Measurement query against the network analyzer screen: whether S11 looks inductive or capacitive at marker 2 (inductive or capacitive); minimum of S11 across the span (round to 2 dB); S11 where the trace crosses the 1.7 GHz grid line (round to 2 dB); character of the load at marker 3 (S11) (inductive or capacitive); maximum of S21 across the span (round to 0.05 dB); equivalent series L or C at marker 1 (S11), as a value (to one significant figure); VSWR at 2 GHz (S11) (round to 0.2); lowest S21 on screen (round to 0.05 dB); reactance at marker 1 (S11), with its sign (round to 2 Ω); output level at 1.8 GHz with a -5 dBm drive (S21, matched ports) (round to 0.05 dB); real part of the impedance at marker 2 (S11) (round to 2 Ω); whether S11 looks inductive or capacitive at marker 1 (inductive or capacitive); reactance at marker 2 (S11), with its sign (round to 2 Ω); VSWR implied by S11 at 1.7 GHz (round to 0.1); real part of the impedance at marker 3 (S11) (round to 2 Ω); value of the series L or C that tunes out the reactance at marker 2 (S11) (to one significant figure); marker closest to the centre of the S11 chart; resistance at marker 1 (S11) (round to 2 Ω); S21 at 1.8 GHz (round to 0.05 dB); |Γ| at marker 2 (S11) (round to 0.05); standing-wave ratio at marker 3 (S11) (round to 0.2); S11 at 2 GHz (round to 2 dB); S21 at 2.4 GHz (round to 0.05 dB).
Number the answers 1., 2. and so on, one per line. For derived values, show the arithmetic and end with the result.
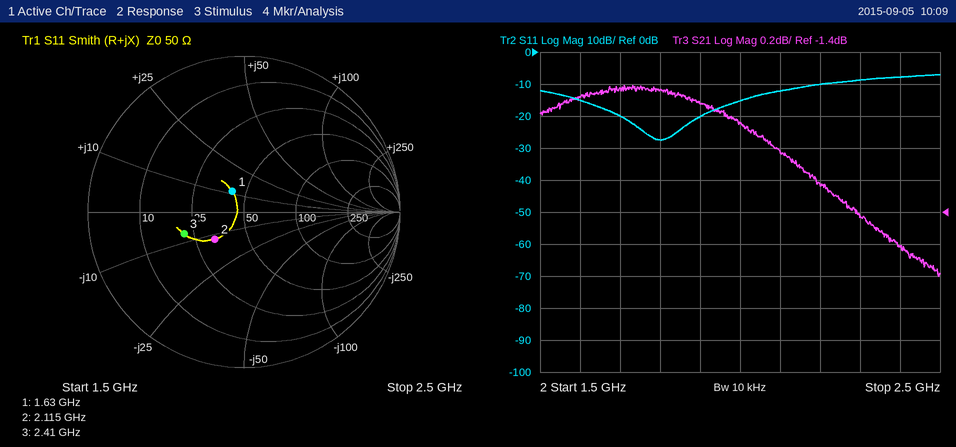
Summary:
1. capacitive
2. -28 dB
3. -20 dB
4. capacitive
5. -0.60 dB
6. L = 12 Ω/(2π × 1.63 GHz) ≈ 1 nH
7. |Γ| = 10^(-16/20) = 0.1585; VSWR = (1 + 0.1585)/(1 − 0.1585) ≈ 1.4
8. -1.80 dB
9. +12 Ω
10. -5 dBm + (-0.65 dB) = -5.65 dBm
11. 32 Ω
12. inductive
13. -12 Ω
14. |Γ| = 10^(-20/20) = 0.1000; VSWR = (1 + 0.1000)/(1 − 0.1000) ≈ 1.2
15. 22 Ω
16. L = 12 Ω/(2π × 2.115 GHz) ≈ 903 pH, so 900 pH to one significant figure
17. marker 1
18. 42 Ω
19. -0.65 dB
20. 0.25
21. 2.4
22. -16 dB
23. -1.60 dB
